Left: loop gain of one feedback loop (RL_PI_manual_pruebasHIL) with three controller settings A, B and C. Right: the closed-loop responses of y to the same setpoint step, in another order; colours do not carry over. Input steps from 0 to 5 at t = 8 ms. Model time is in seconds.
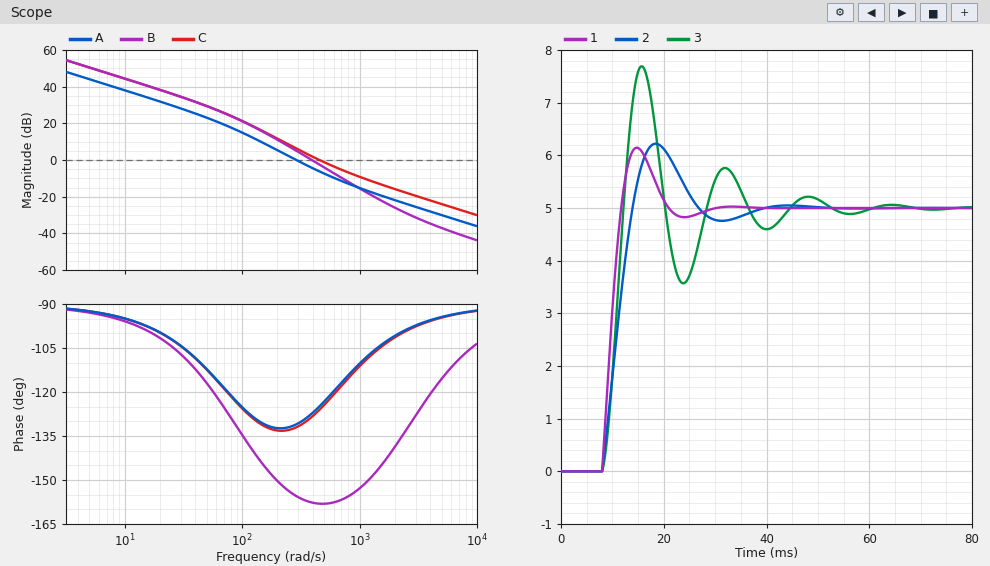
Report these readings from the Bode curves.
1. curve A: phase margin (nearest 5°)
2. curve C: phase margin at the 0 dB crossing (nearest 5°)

50°
55°
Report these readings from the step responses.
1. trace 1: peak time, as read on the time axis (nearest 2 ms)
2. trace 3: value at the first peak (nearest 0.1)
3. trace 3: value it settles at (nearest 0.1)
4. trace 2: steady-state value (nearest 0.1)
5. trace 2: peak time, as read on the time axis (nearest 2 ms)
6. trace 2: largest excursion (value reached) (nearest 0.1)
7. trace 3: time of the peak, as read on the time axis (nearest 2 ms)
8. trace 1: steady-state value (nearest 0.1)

14 ms
7.7
5.0
5.0
18 ms
6.2
16 ms
5.0
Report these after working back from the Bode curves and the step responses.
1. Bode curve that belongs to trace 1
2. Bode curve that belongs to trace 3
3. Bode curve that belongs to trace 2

C
B
A
